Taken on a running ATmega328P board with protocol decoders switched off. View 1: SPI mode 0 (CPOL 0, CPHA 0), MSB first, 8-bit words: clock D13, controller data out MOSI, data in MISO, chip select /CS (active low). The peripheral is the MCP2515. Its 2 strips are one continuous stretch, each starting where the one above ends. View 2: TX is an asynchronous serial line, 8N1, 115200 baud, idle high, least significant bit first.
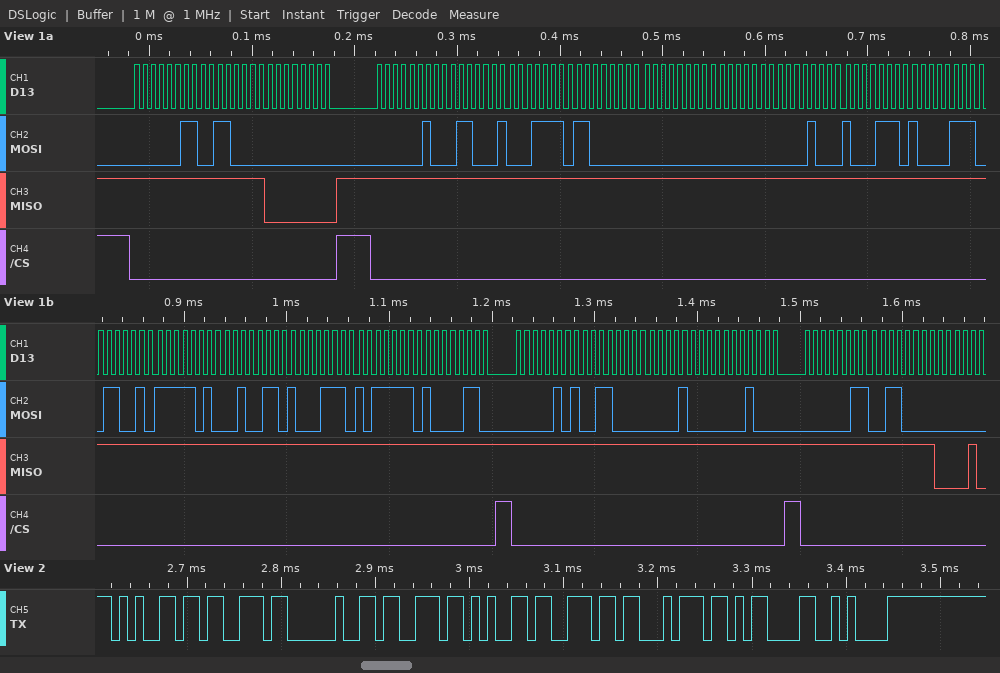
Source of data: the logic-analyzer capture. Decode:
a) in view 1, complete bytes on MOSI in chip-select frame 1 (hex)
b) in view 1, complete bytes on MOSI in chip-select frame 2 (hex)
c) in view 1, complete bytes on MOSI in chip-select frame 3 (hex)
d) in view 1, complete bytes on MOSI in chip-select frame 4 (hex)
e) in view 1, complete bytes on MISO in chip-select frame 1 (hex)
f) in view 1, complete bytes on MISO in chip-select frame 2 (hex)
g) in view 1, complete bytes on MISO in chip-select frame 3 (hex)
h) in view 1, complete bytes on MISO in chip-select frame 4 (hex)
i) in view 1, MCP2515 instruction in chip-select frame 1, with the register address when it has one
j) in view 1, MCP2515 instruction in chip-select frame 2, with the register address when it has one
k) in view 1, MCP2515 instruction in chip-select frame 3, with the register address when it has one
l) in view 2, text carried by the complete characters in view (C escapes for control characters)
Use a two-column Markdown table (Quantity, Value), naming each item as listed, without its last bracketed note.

| Quantity | Value |
|---|---|
| in view 1, complete bytes on MOSI in chip-select frame 1 | 03 30 00 |
| in view 1, complete bytes on MOSI in chip-select frame 2 | 02 31 1E C0 00 00 08 8E 87 32 FA 26 8E BE 86 |
| in view 1, complete bytes on MOSI in chip-select frame 3 | 05 30 08 08 |
| in view 1, complete bytes on MOSI in chip-select frame 4 | 03 30 |
| in view 1, complete bytes on MISO in chip-select frame 1 | FF FF 00 |
| in view 1, complete bytes on MISO in chip-select frame 2 | FF FF FF FF FF FF FF FF FF FF FF FF FF FF FF |
| in view 1, complete bytes on MISO in chip-select frame 3 | FF FF FF FF |
| in view 1, complete bytes on MISO in chip-select frame 4 | FF FF |
| in view 1, MCP2515 instruction in chip-select frame 1, with the register address when it has one | READ 0x30 |
| in view 1, MCP2515 instruction in chip-select frame 2, with the register address when it has one | WRITE 0x31 |
| in view 1, MCP2515 instruction in chip-select frame 3, with the register address when it has one | BIT MODIFY 0x30 |
| in view 2, text carried by the complete characters in view | "es sent\r\n" |
